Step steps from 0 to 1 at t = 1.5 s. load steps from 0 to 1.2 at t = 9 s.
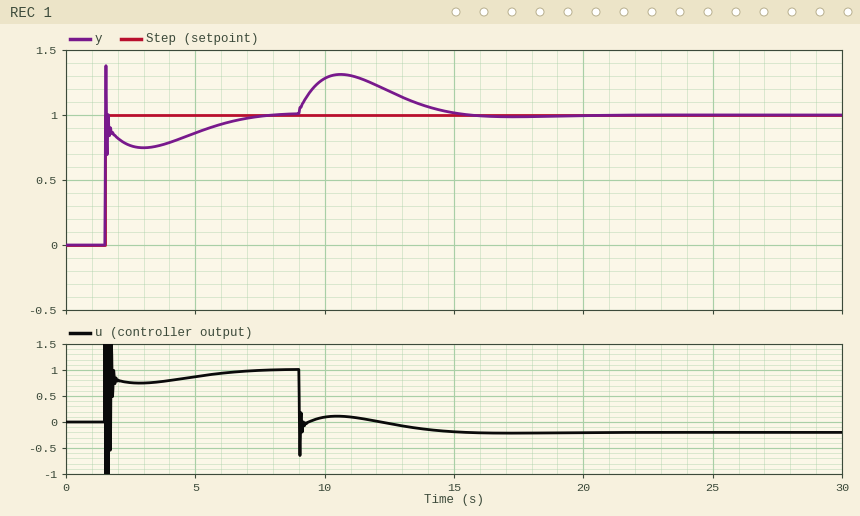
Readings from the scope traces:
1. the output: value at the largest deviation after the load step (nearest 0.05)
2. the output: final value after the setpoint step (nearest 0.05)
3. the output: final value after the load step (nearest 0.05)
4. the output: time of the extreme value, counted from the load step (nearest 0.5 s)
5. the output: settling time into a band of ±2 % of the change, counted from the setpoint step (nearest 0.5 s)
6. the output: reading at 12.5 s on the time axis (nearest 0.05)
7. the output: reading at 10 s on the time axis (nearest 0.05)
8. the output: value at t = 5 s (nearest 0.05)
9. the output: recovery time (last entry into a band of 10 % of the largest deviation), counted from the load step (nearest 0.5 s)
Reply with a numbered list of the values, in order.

1. 1.30
2. 1.00
3. 1.00
4. 1.5 s
5. 5.5 s
6. 1.20
7. 1.30
8. 0.85
9. 5.5 s
